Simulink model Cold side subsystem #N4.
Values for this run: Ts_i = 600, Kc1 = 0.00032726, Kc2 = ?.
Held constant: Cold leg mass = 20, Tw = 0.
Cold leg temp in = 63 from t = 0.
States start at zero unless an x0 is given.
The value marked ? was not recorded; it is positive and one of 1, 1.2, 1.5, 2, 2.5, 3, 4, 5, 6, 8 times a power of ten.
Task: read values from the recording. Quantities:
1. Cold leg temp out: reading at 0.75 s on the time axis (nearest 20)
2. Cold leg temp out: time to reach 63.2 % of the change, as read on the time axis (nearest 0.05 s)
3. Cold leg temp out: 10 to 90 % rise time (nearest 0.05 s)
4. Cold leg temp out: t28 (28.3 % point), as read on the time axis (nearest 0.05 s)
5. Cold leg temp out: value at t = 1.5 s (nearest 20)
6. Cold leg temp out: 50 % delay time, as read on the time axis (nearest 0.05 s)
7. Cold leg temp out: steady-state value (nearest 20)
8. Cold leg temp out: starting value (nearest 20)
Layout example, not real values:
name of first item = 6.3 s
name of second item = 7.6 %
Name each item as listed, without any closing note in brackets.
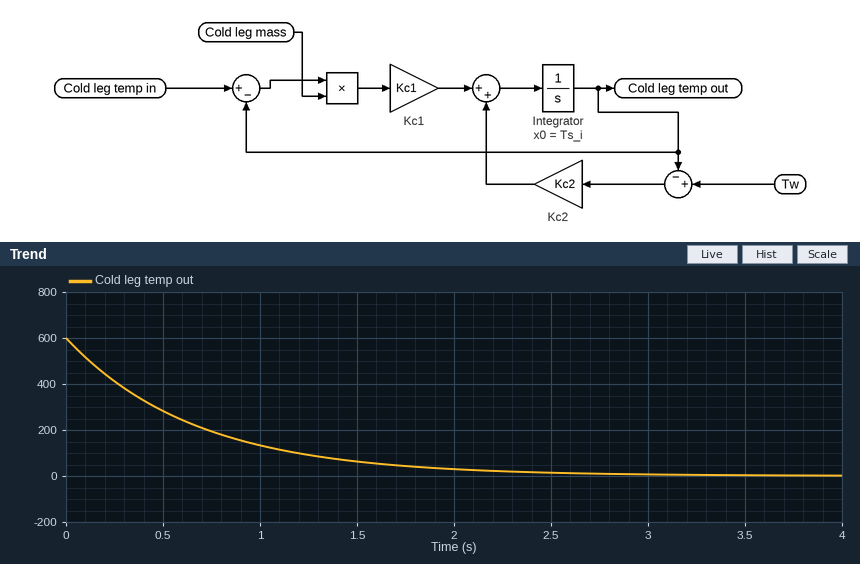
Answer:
Cold leg temp out: reading at 0.75 s on the time axis = 200
Cold leg temp out: time to reach 63.2 % of the change, as read on the time axis = 0.65 s
Cold leg temp out: 10 to 90 % rise time = 1.45 s
Cold leg temp out: t28 (28.3 % point), as read on the time axis = 0.20 s
Cold leg temp out: value at t = 1.5 s = 60
Cold leg temp out: 50 % delay time, as read on the time axis = 0.45 s
Cold leg temp out: steady-state value = 0
Cold leg temp out: starting value = 600
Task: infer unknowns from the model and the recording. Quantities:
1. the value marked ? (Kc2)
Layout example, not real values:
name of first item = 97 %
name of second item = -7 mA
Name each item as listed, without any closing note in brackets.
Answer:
the value marked ? = 1.5
